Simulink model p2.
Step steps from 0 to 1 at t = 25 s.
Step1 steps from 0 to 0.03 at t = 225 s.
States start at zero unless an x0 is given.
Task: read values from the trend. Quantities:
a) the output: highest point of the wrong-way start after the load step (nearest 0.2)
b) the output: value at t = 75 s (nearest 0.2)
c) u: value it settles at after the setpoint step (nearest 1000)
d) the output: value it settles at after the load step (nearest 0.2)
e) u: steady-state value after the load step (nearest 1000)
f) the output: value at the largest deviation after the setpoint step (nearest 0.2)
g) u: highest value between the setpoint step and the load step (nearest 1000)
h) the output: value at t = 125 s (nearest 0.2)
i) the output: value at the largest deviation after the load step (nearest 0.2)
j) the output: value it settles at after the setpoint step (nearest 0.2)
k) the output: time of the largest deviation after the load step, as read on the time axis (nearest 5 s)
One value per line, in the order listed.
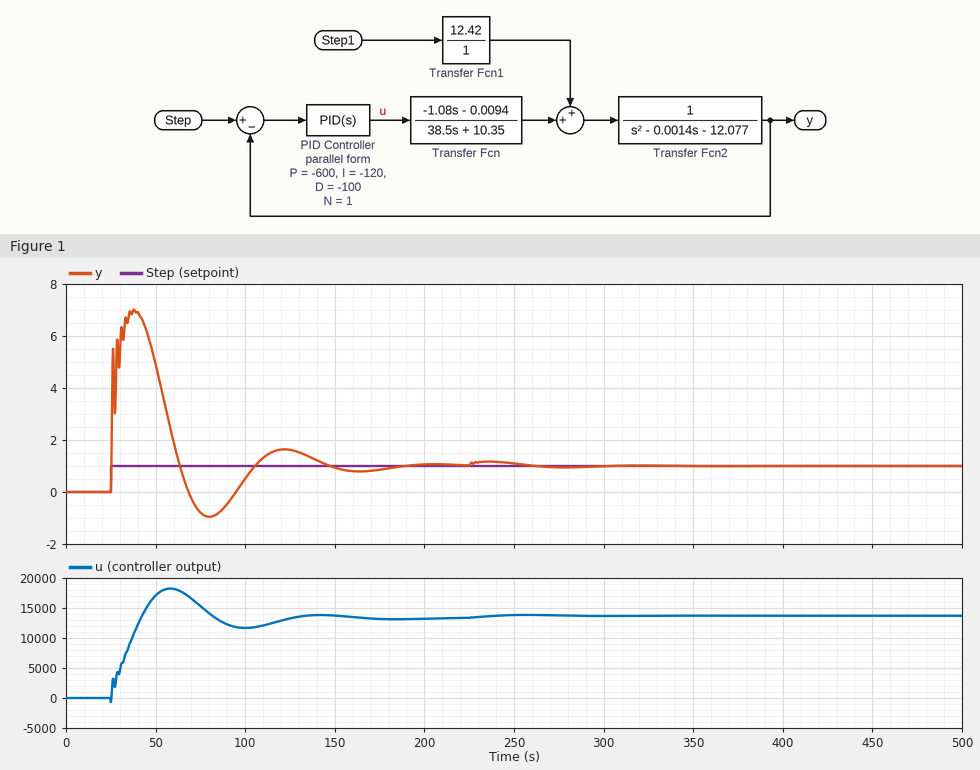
1.2
-0.8
13000
1.0
14000
7.0
18000
1.6
1.0
1.0
280 s
